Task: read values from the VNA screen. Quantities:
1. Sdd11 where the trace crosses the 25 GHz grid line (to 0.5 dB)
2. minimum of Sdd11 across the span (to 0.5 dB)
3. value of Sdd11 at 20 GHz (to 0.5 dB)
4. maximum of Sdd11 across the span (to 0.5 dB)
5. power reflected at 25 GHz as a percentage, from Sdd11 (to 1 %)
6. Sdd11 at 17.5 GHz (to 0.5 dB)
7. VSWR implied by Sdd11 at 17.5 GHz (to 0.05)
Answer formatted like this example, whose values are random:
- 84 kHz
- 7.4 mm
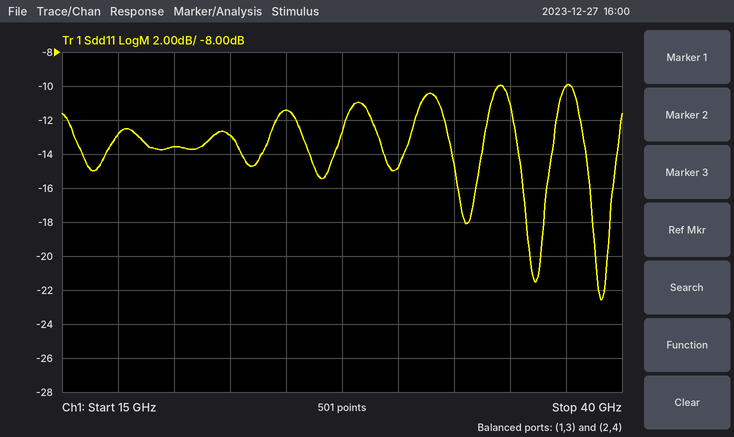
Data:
- -11.5 dB
- -22.5 dB
- -13.5 dB
- -10.0 dB
- 7 %
- -13.0 dB
- 1.60
